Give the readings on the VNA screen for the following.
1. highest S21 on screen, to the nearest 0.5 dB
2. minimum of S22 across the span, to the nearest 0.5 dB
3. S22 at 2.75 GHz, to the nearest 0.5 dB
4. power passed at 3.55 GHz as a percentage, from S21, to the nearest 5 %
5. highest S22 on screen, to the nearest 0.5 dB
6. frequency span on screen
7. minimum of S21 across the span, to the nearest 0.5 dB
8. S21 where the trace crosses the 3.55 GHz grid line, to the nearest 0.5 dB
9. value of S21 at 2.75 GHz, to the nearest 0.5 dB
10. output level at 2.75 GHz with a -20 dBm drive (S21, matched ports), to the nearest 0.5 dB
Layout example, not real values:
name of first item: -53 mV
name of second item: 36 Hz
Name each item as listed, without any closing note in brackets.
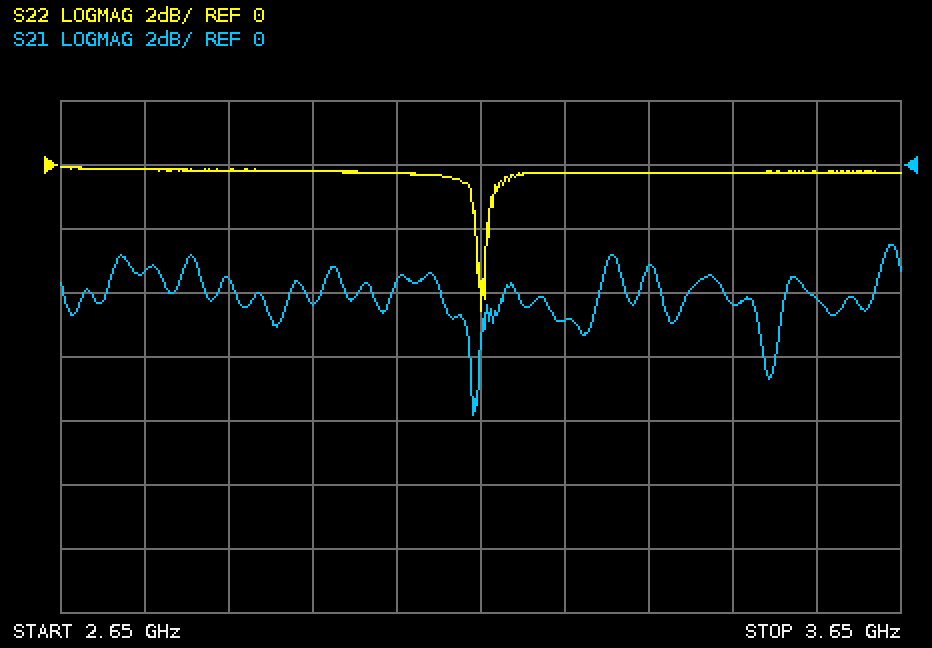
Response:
highest S21 on screen, to the nearest 0.5 dB: -2.5 dB
minimum of S22 across the span, to the nearest 0.5 dB: -4.5 dB
S22 at 2.75 GHz, to the nearest 0.5 dB: 0.0 dB
power passed at 3.55 GHz as a percentage, from S21, to the nearest 5 %: 40 %
highest S22 on screen, to the nearest 0.5 dB: 0.0 dB
frequency span on screen: 1 GHz
minimum of S21 across the span, to the nearest 0.5 dB: -8.0 dB
S21 where the trace crosses the 3.55 GHz grid line, to the nearest 0.5 dB: -4.0 dB
value of S21 at 2.75 GHz, to the nearest 0.5 dB: -3.5 dB
output level at 2.75 GHz with a -20 dBm drive (S21, matched ports), to the nearest 0.5 dB: -23.5 dBm
